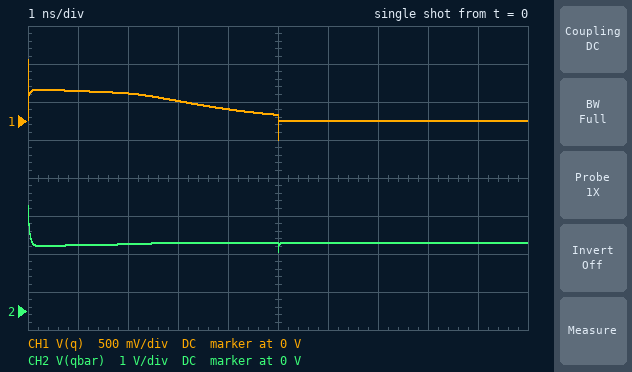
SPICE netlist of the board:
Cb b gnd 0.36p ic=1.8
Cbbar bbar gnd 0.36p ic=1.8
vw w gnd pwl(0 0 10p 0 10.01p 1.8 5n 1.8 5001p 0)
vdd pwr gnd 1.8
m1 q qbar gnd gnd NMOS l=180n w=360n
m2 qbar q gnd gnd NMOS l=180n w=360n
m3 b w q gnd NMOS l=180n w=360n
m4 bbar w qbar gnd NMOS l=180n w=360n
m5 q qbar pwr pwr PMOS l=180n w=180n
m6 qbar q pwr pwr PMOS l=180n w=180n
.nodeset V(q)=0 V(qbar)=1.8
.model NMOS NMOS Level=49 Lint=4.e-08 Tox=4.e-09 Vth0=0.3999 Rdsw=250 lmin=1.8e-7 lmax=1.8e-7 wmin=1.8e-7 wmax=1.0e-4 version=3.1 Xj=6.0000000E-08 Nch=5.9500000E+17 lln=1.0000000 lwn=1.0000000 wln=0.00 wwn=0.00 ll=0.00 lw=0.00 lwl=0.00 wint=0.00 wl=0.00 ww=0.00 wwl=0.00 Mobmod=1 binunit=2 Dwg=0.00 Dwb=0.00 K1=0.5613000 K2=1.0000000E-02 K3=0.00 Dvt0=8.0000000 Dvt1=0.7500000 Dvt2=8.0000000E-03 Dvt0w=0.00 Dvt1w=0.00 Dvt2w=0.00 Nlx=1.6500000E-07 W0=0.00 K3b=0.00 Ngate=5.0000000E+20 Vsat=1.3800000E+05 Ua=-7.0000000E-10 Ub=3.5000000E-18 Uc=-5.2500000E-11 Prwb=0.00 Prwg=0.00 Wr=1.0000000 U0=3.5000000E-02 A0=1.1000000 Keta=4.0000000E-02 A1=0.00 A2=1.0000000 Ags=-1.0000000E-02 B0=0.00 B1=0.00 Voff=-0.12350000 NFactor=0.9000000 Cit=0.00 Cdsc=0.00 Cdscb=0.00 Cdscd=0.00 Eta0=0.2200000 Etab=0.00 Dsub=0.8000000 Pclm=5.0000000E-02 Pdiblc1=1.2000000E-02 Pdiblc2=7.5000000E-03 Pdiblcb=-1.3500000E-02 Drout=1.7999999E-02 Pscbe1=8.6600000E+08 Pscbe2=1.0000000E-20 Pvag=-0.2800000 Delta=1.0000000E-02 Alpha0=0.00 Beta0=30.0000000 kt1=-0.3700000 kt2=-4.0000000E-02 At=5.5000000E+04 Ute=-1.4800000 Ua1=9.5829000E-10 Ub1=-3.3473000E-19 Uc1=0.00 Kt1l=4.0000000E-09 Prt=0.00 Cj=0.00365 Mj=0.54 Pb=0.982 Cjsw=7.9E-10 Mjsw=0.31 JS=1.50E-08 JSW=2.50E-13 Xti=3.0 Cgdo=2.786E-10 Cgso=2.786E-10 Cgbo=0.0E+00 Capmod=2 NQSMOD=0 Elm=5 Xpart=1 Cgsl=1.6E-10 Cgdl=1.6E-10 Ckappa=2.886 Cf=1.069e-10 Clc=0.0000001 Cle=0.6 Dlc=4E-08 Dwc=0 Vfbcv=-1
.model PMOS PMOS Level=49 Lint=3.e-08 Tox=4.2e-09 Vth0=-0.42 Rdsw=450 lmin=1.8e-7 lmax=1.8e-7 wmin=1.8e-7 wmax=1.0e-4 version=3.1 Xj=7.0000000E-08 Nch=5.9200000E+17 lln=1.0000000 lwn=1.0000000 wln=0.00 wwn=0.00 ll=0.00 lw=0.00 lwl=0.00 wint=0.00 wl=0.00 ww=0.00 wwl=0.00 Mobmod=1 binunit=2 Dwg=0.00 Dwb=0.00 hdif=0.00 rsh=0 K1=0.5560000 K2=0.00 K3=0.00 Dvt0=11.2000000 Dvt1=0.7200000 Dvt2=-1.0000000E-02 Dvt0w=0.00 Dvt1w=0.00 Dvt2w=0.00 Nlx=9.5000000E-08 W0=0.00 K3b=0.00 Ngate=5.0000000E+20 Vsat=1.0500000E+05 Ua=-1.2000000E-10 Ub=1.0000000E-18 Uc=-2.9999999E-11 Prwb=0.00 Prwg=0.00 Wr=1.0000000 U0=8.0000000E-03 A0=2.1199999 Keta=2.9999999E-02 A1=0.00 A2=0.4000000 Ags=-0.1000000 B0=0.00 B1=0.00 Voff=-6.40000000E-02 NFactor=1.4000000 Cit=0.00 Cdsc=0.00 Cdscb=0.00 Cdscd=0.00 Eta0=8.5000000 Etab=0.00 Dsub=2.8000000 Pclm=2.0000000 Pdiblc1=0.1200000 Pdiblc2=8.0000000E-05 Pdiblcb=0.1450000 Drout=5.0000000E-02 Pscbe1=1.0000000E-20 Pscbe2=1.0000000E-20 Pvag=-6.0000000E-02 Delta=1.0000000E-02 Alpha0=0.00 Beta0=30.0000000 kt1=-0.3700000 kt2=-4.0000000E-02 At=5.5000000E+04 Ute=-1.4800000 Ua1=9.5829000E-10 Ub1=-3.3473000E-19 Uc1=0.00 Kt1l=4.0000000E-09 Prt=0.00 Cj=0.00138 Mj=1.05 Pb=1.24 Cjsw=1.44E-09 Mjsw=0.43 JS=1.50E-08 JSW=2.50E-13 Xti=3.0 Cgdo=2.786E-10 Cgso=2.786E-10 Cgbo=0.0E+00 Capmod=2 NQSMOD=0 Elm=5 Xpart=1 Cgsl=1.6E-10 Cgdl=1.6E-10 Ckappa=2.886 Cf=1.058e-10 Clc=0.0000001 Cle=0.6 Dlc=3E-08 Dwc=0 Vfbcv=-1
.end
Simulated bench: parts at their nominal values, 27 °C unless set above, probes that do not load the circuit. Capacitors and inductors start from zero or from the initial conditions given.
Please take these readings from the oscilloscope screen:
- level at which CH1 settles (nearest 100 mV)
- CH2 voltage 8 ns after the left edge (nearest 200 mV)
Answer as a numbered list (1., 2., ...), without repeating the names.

1. 0 V
2. 1.8 V
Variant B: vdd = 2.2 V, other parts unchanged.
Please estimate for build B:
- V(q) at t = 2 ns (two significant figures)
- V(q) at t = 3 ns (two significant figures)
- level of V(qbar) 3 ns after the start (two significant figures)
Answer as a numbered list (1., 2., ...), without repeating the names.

1. 330 mV
2. 230 mV
3. 2.2 V
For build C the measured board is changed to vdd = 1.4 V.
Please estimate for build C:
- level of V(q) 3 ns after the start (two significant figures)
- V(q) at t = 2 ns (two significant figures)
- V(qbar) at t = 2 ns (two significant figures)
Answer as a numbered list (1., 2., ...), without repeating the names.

1. 760 mV
2. 790 mV
3. 880 mV
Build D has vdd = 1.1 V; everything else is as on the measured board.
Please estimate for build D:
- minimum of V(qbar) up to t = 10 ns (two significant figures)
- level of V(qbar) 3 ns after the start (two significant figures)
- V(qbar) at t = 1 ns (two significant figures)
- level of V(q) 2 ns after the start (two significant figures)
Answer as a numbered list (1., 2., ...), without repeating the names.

1. 630 mV
2. 840 mV
3. 850 mV
4. 810 mV
